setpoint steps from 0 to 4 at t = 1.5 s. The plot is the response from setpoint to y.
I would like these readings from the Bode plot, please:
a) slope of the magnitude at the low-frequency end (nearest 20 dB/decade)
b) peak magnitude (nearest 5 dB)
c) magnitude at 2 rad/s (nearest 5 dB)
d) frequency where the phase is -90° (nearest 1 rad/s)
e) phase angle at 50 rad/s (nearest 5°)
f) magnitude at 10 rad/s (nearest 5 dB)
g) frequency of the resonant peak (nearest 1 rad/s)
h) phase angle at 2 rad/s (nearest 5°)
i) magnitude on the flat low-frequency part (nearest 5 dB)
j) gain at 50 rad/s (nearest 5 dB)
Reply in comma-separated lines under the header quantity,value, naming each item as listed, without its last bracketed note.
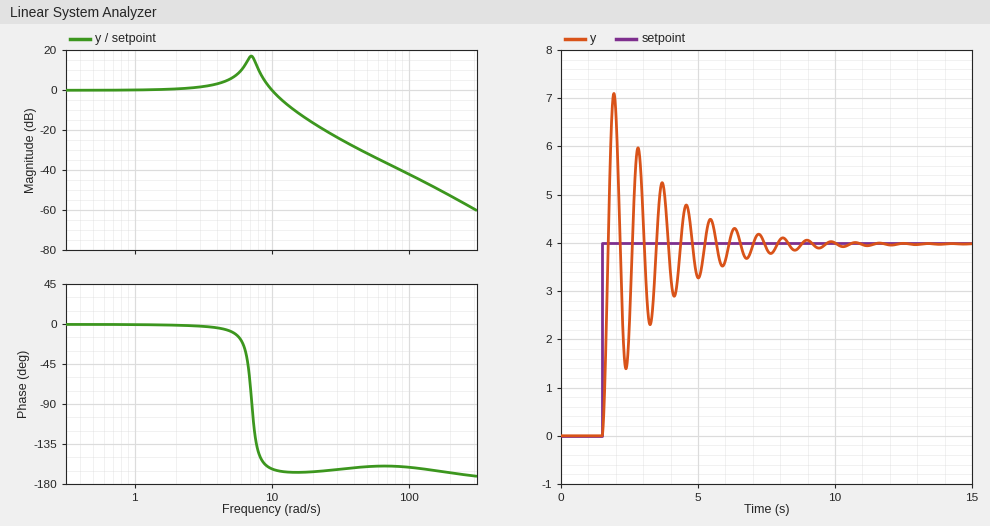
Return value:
quantity,value
slope of the magnitude at the low-frequency end,0 dB/decade
peak magnitude,15 dB
magnitude at 2 rad/s,0 dB
frequency where the phase is -90°,7 rad/s
phase angle at 50 rad/s,-160°
magnitude at 10 rad/s,0 dB
frequency of the resonant peak,7 rad/s
phase angle at 2 rad/s,0°
magnitude on the flat low-frequency part,0 dB
gain at 50 rad/s,-30 dB
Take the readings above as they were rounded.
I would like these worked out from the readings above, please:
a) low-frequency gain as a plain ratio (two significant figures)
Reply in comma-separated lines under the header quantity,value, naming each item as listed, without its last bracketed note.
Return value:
quantity,value
low-frequency gain as a plain ratio,1.0
